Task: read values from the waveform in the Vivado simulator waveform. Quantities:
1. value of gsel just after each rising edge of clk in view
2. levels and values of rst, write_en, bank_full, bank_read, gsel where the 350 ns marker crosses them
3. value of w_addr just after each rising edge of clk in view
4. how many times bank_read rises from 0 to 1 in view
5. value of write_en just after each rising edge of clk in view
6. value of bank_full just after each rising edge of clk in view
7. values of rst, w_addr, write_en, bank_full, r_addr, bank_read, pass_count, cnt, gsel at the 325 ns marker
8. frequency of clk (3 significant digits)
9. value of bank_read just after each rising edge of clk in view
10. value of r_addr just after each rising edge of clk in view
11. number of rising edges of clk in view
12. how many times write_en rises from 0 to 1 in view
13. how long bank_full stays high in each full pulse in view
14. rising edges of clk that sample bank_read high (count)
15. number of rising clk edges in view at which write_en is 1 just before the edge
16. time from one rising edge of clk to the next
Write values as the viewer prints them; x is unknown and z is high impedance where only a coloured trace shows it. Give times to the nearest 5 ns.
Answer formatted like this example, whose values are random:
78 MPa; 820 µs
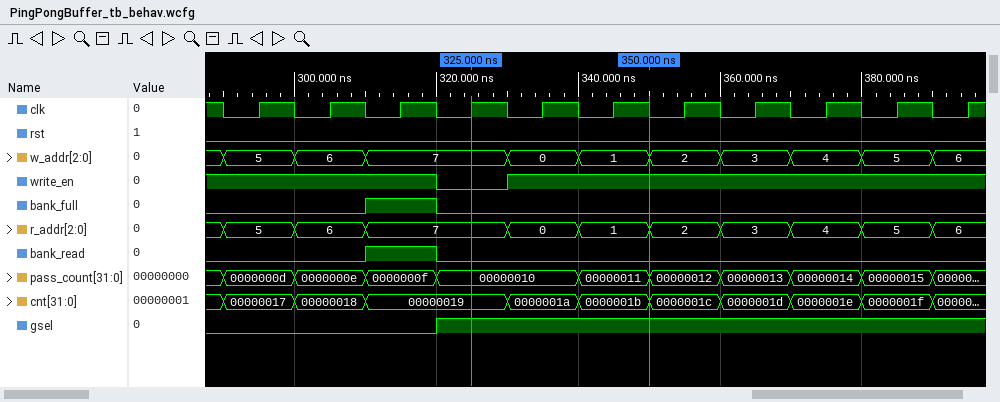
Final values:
0 0 0 1 1 1 1 1 1 1 1; rst=0, write_en=1, bank_full=0, bank_read=0, gsel=1; 5, 6, 7, 7, 0, 1, 2, 3, 4, 5, 6; 1; 1 1 1 0 1 1 1 1 1 1 1; 0 0 1 0 0 0 0 0 0 0 0; rst=0, w_addr=7, write_en=0, bank_full=0, r_addr=7, bank_read=0, pass_count=00000010, cnt=00000019, gsel=1; 100 MHz; 0 0 1 0 0 0 0 0 0 0 0; 5, 6, 7, 7, 0, 1, 2, 3, 4, 5, 6; 11; 1; 10 ns; 1; 10; 10 ns
